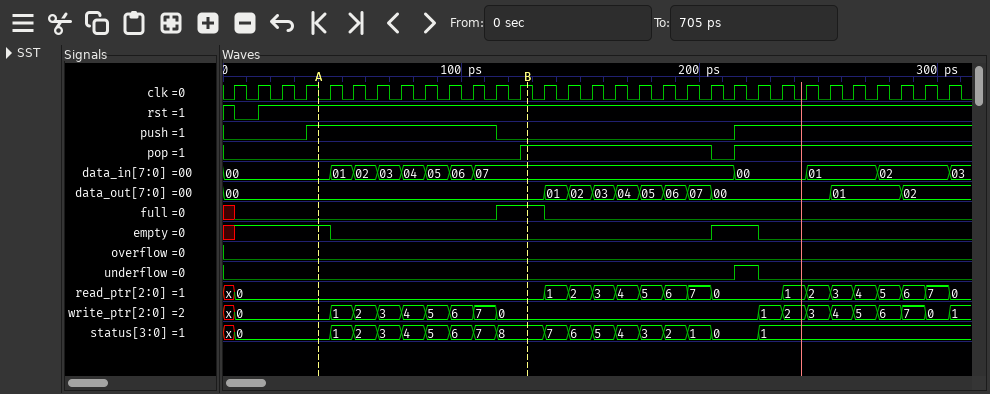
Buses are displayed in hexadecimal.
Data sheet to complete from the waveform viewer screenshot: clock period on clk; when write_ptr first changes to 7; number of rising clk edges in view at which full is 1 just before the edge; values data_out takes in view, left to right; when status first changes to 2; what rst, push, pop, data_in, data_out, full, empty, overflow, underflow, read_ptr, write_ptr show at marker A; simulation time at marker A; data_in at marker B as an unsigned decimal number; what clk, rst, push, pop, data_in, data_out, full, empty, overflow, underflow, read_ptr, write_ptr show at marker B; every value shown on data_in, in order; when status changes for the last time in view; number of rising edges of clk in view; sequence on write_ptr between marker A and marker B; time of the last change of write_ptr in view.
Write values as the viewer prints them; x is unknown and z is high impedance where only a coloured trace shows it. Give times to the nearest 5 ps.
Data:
10 ps
105 ps
2
00, 01, 02, 03, 04, 05, 06, 07, 00, 01, 02
55 ps
rst=1, push=1, pop=0, data_in=00, data_out=00, full=0, empty=1, overflow=0, underflow=0, read_ptr=0, write_ptr=0
40 ps
7
clk=1, rst=1, push=0, pop=1, data_in=07, data_out=00, full=1, empty=0, overflow=0, underflow=0, read_ptr=0, write_ptr=0
00, 01, 02, 03, 04, 05, 06, 07, 00, 01, 02, 03
225 ps
31
0, 1, 2, 3, 4, 5, 6, 7, 0
305 ps
